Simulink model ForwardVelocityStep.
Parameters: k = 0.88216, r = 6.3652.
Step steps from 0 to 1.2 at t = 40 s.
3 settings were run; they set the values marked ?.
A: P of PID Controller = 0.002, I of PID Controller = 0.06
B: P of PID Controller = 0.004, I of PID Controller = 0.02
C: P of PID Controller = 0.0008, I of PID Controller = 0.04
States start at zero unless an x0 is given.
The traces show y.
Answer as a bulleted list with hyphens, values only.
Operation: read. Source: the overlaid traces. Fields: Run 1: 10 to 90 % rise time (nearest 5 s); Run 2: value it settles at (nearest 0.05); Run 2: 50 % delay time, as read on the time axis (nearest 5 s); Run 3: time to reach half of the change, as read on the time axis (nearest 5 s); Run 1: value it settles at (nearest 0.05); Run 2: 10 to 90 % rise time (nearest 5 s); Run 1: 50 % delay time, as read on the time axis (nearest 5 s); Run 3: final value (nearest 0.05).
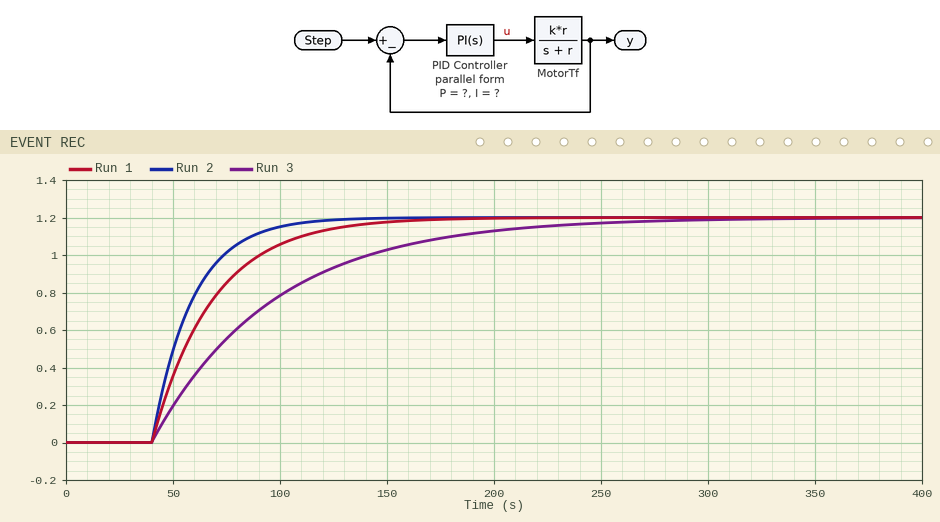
- 60 s
- 1.20
- 55 s
- 80 s
- 1.20
- 40 s
- 60 s
- 1.20
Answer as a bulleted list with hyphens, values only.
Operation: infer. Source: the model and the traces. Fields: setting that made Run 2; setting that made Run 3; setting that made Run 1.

- A
- B
- C
